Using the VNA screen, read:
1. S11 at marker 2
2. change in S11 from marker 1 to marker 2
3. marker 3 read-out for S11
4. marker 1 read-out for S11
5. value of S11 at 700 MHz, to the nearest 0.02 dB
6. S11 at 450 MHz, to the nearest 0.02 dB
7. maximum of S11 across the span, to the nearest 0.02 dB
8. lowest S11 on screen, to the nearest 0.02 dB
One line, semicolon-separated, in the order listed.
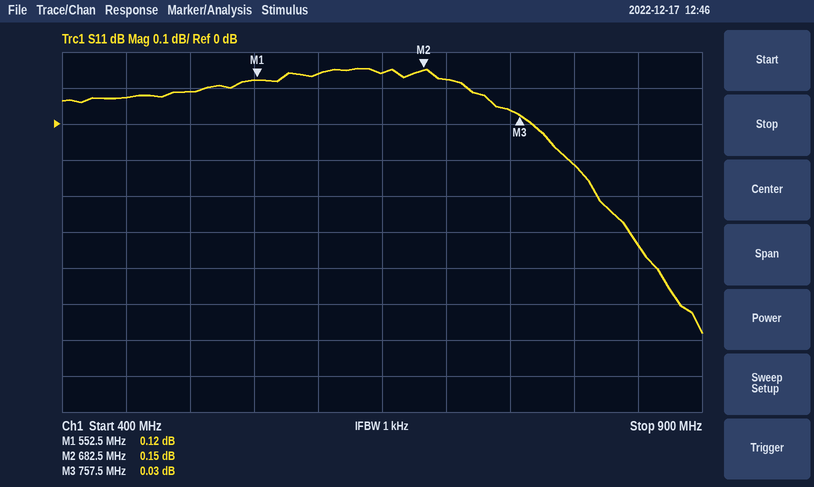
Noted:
0.15 dB; 0.03 dB; 0.03 dB; 0.12 dB; 0.12 dB; 0.08 dB; 0.16 dB; -0.58 dB
